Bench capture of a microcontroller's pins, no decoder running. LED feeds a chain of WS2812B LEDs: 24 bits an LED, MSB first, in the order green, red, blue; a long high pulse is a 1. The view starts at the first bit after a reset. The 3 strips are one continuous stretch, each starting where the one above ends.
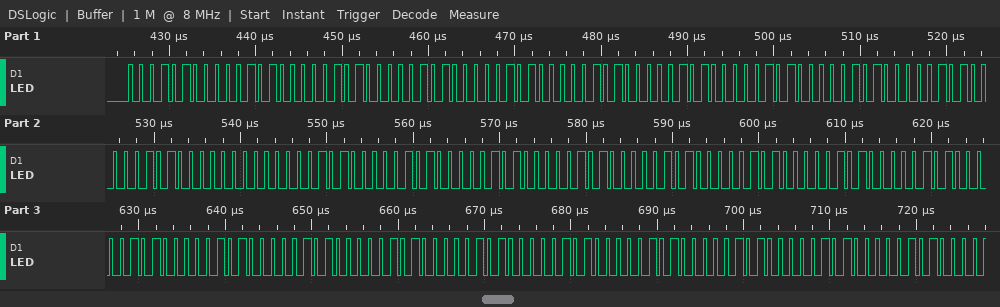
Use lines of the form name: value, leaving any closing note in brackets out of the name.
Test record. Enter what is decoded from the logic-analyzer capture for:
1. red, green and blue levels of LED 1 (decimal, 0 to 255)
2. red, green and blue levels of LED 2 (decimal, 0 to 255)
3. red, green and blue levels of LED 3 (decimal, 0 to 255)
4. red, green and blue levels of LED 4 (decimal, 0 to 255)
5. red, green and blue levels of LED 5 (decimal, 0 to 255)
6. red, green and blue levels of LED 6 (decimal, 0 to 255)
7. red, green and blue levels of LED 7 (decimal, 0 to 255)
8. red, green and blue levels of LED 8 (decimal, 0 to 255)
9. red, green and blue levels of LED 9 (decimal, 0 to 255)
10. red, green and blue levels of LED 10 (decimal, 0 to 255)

red, green and blue levels of LED 1: 20, 20, 20
red, green and blue levels of LED 2: 20, 20, 20
red, green and blue levels of LED 3: 20, 20, 20
red, green and blue levels of LED 4: 20, 20, 0
red, green and blue levels of LED 5: 20, 20, 20
red, green and blue levels of LED 6: 20, 20, 20
red, green and blue levels of LED 7: 20, 20, 20
red, green and blue levels of LED 8: 20, 20, 20
red, green and blue levels of LED 9: 20, 20, 20
red, green and blue levels of LED 10: 20, 20, 20
